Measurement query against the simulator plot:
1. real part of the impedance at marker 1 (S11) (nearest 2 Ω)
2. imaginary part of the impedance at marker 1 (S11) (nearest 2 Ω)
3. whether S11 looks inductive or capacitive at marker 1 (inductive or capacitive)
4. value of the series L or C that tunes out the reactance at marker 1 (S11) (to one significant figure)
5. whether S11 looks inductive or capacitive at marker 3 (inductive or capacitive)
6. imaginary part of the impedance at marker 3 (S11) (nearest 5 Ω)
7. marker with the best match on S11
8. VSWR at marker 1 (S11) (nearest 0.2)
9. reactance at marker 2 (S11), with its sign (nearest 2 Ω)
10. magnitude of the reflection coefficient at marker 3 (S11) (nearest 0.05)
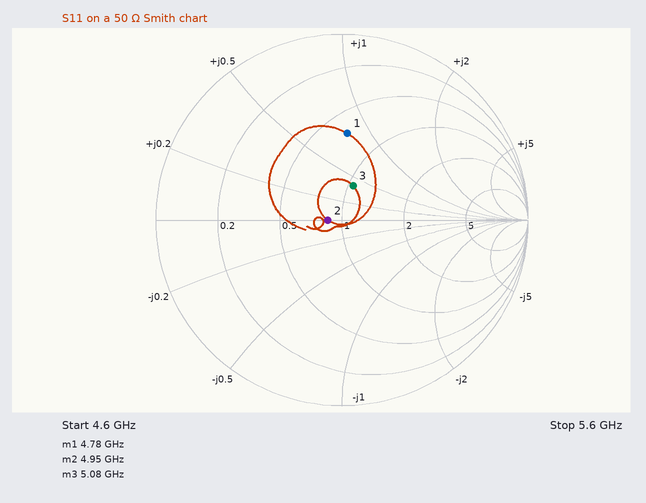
34 Ω
+40 Ω
inductive
800 fF
inductive
+20 Ω
marker 2
2.8
0 Ω
0.20
